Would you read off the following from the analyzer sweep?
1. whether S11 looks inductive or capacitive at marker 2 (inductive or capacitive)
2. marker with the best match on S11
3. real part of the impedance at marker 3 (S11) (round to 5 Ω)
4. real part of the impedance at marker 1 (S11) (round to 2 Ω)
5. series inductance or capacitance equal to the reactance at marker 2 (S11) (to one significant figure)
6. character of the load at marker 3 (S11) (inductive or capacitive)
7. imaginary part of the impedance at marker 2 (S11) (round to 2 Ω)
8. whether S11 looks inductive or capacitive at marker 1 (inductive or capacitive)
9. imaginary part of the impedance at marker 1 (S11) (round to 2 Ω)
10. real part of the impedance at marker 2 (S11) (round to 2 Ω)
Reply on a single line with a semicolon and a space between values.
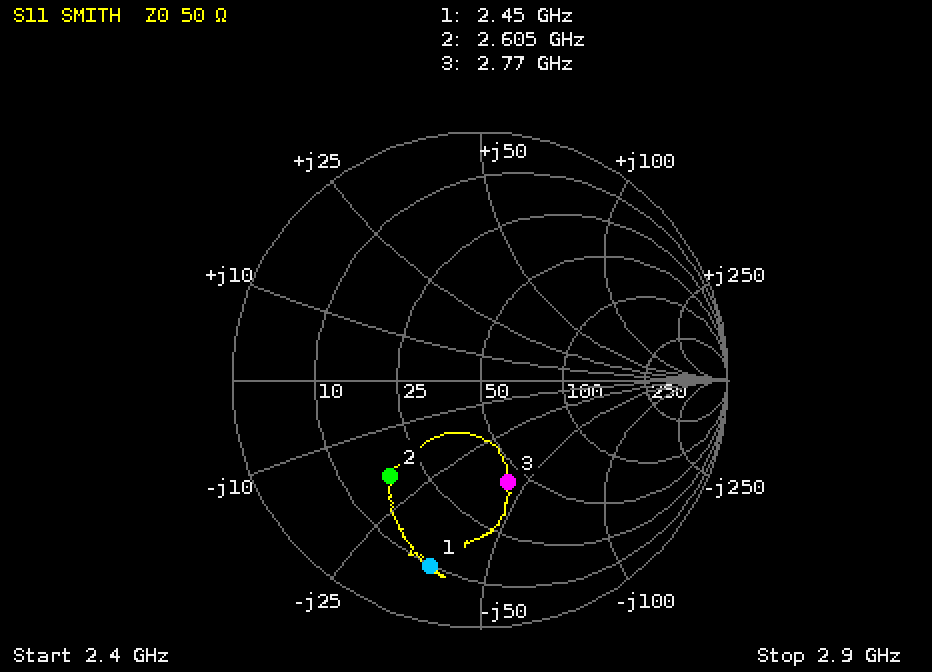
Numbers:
capacitive; marker 3; 45 Ω; 10 Ω; 3 pF; capacitive; -20 Ω; capacitive; -38 Ω; 18 Ω
